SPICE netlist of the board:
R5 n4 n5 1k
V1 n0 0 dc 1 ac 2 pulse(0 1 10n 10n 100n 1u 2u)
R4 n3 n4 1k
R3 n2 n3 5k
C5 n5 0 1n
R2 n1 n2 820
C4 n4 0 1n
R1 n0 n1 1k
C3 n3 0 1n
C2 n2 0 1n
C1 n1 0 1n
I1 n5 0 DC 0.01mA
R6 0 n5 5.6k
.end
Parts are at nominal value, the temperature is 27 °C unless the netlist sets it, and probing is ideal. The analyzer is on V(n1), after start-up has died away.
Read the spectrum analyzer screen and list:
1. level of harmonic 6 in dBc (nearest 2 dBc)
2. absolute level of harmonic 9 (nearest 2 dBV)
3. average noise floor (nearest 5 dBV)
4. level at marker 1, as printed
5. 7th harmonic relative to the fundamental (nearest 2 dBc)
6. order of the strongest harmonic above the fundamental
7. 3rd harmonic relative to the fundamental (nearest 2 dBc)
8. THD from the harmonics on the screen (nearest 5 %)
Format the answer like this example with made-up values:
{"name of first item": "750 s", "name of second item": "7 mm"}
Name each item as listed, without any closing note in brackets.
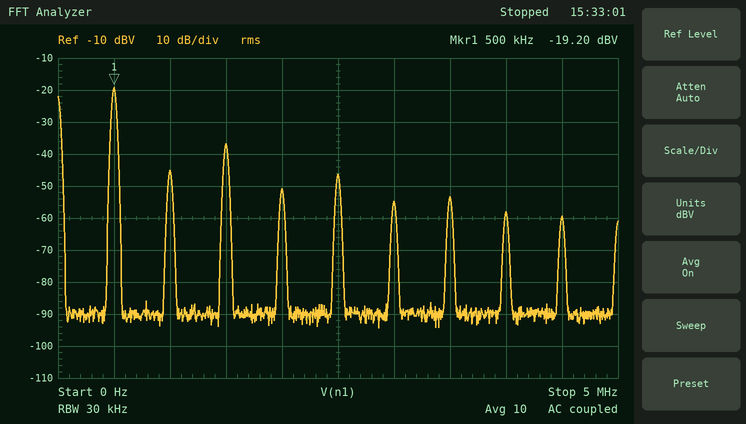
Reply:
{"level of harmonic 6 in dBc": "-36 dBc", "absolute level of harmonic 9": "-60 dBV", "average noise floor": "-90 dBV", "level at marker 1, as printed": "-19.20 dBV", "7th harmonic relative to the fundamental": "-34 dBc", "order of the strongest harmonic above the fundamental": "3", "3rd harmonic relative to the fundamental": "-18 dBc", "THD from the harmonics on the screen": "15 %"}
